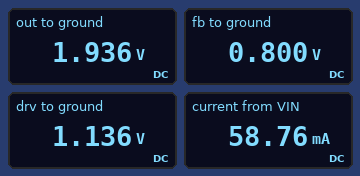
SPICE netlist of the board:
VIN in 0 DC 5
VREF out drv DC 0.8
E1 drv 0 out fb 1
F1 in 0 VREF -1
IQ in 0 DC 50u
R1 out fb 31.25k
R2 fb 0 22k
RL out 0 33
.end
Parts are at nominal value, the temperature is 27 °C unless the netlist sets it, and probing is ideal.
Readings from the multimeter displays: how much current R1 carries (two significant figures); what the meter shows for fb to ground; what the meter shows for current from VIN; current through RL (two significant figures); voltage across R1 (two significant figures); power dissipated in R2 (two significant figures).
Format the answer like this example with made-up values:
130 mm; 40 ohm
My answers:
36 µA; 0.800 V; 58.76 mA; 59 mA; 1.1 V; 29 µW
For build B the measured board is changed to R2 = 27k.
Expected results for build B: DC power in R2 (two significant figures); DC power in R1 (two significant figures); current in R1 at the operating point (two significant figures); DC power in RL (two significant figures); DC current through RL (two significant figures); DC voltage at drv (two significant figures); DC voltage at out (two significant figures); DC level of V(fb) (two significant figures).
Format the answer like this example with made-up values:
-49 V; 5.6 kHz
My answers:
24 µW; 27 µW; 30 µA; 90 mW; 52 mA; 930 mV; 1.7 V; 800 mV
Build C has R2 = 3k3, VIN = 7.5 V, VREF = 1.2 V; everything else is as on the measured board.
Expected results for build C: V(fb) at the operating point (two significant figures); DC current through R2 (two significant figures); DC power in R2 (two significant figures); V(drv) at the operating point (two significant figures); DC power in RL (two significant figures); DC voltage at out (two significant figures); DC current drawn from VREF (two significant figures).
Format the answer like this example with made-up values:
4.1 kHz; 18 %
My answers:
1.2 V; 360 µA; 440 µW; 11 V; 4.8 W; 13 V; 380 mA
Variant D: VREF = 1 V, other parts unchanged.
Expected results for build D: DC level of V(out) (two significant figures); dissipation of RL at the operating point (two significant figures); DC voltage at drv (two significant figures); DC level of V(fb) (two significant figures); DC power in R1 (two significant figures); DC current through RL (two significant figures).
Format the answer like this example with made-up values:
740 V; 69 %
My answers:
2.4 V; 180 mW; 1.4 V; 1.0 V; 65 µW; 73 mA
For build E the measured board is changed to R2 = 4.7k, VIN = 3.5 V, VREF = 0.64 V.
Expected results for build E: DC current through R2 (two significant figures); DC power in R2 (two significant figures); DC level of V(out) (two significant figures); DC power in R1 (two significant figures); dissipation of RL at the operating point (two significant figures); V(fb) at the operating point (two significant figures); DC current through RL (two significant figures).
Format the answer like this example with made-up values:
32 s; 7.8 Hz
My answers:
140 µA; 87 µW; 4.9 V; 580 µW; 730 mW; 640 mV; 150 mA
